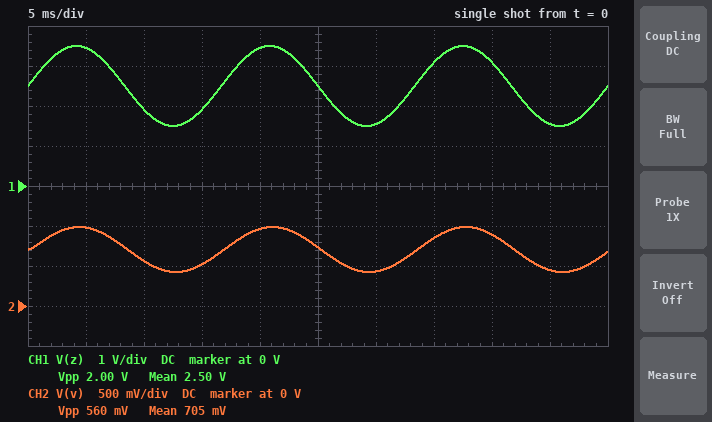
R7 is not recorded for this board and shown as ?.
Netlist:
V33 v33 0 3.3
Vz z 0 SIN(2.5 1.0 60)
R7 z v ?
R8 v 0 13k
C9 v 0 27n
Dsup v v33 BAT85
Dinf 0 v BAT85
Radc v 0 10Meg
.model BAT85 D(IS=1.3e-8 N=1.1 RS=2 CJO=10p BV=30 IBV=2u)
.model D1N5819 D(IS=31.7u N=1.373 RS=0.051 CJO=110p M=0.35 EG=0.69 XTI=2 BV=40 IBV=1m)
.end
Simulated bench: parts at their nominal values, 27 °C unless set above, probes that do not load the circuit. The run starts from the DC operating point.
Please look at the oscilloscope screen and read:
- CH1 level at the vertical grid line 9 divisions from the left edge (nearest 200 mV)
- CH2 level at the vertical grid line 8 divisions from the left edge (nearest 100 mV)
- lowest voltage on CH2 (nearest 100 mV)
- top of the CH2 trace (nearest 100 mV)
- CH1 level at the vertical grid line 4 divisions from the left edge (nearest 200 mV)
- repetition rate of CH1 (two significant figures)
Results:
1.6 V
900 mV
400 mV
1.0 V
3.4 V
60 Hz
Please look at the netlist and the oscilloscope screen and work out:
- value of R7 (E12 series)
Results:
33 kΩ
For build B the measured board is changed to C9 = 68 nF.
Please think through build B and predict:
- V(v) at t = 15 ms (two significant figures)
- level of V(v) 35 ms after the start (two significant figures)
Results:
500 mV
810 mV
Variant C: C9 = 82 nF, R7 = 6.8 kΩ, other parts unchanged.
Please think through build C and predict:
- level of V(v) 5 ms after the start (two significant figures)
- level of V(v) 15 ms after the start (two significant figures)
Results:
2.3 V
1.2 V
